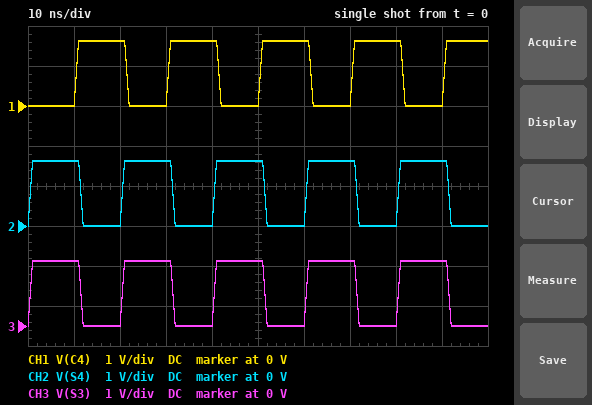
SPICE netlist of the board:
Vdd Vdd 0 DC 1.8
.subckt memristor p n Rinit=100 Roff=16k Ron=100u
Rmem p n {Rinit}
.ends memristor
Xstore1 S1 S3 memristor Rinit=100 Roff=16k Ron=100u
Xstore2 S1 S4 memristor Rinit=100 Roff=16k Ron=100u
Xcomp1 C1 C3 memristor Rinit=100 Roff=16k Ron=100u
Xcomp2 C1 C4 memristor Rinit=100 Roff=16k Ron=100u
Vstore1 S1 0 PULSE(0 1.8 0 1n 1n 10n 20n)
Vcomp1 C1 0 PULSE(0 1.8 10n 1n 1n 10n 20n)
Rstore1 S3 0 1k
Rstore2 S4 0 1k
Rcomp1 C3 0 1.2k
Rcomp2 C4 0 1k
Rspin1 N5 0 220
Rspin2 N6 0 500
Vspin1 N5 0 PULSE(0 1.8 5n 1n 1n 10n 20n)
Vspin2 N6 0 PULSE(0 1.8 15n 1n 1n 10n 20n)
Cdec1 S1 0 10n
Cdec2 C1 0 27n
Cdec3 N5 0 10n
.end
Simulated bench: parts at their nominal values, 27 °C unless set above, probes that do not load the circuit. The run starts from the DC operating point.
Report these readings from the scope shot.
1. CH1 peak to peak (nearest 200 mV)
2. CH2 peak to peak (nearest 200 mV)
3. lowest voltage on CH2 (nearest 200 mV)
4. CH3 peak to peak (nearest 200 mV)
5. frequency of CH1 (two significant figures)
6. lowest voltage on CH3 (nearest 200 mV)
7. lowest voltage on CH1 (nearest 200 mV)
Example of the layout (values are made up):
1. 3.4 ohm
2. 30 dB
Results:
1. 1.6 V
2. 1.6 V
3. 0 V
4. 1.6 V
5. 50 MHz
6. 0 V
7. 0 V
